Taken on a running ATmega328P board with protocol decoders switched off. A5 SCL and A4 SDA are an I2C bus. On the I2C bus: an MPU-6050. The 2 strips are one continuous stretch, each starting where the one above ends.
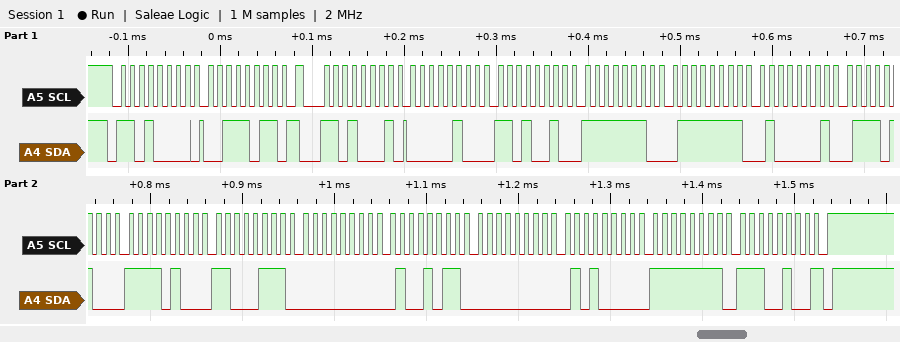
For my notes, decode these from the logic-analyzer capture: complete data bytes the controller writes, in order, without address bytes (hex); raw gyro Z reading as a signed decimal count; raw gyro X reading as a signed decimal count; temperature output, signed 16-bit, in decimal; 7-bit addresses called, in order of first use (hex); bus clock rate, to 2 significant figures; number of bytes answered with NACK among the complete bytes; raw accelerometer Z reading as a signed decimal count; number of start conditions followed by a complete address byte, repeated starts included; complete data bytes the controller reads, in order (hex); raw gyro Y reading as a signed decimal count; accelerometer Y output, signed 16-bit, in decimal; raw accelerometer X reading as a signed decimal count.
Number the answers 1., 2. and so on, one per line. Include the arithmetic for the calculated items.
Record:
1. 3B
2. 0xFFE4 = -28
3. 0x004B = 75
4. 0xF4C7 = -2873
5. 0x68
6. 100 kHz
7. 1
8. 0x4174 = 16756
9. 2
10. 04 D2 FE 7F 41 74 F4 C7 00 4B 00 50 FF E4
11. 0x0050 = 80
12. 0xFE7F = -385
13. 0x04D2 = 1234
